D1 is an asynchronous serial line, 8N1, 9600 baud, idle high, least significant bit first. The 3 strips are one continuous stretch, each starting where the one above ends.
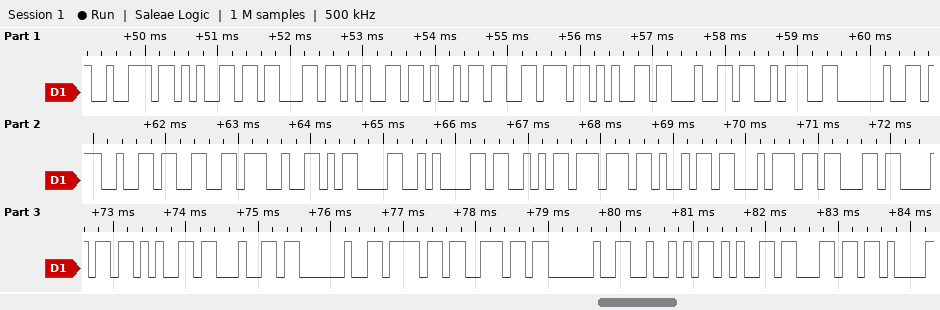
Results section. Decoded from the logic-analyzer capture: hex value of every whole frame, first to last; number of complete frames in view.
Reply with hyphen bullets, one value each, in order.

- 72 65 63 65 69 76 65 64 3A 20 27 33 27 0D 0A 53 77 69 74 63 68 65 64 20 6F 6E 20 52 65 6C
- 30
